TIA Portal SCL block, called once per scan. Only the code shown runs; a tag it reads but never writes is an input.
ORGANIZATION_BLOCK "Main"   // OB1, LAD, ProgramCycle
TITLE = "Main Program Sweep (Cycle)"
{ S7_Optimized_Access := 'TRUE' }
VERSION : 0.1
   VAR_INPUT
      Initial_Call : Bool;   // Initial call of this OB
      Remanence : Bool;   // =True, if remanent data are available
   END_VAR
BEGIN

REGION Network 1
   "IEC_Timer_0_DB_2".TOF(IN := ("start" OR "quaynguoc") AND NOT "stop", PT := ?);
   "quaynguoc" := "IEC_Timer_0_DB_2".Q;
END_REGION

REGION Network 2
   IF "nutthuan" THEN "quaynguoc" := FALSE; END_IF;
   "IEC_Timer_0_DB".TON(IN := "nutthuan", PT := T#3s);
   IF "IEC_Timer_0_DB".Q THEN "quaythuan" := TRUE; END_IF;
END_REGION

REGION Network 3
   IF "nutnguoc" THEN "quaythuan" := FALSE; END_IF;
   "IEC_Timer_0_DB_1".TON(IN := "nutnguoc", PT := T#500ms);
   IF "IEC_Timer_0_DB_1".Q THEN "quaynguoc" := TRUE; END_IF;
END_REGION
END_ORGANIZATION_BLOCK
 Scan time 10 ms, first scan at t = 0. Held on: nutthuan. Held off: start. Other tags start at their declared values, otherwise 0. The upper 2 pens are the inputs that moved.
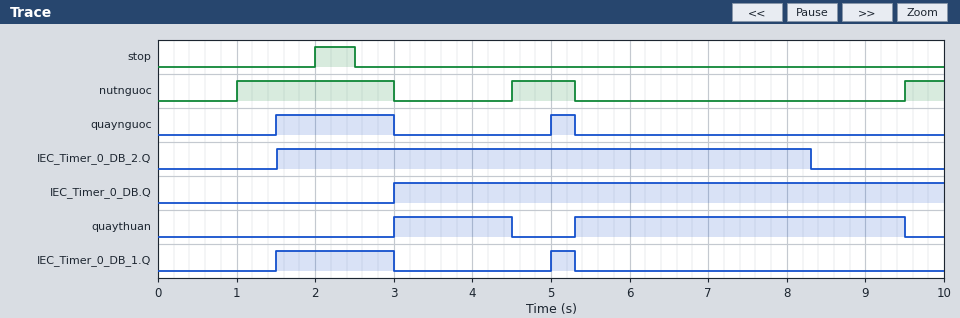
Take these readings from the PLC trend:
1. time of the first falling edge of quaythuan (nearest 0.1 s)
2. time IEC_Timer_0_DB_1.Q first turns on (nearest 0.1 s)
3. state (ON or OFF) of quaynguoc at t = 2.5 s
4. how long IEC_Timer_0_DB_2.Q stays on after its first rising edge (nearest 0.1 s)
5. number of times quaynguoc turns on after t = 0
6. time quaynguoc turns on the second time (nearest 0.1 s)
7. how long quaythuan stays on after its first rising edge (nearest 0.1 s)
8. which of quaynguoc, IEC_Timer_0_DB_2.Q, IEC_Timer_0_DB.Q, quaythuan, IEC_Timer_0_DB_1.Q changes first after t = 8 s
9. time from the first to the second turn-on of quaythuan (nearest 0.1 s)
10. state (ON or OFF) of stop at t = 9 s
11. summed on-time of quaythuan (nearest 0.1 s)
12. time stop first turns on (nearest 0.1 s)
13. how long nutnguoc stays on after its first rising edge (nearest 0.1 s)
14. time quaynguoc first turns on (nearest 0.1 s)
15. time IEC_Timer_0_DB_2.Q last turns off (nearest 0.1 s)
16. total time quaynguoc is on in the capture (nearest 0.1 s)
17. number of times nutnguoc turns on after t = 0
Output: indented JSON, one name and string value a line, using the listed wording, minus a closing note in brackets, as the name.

{
  "time of the first falling edge of quaythuan": "4.5 s",
  "time IEC_Timer_0_DB_1.Q first turns on": "1.5 s",
  "state (ON or OFF) of quaynguoc at t = 2.5 s": "ON",
  "how long IEC_Timer_0_DB_2.Q stays on after its first rising edge": "6.8 s",
  "number of times quaynguoc turns on after t = 0": "2",
  "time quaynguoc turns on the second time": "5.0 s",
  "how long quaythuan stays on after its first rising edge": "1.5 s",
  "which of quaynguoc, IEC_Timer_0_DB_2.Q, IEC_Timer_0_DB.Q, quaythuan, IEC_Timer_0_DB_1.Q changes first after t = 8 s": "IEC_Timer_0_DB_2.Q",
  "time from the first to the second turn-on of quaythuan": "2.3 s",
  "state (ON or OFF) of stop at t = 9 s": "OFF",
  "summed on-time of quaythuan": "5.7 s",
  "time stop first turns on": "2.0 s",
  "how long nutnguoc stays on after its first rising edge": "2.0 s",
  "time quaynguoc first turns on": "1.5 s",
  "time IEC_Timer_0_DB_2.Q last turns off": "8.3 s",
  "total time quaynguoc is on in the capture": "1.8 s",
  "number of times nutnguoc turns on after t = 0": "3"
}
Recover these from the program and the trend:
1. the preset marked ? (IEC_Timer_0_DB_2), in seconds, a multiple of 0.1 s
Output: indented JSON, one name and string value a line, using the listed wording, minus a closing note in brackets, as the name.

{
  "the preset marked ? (IEC_Timer_0_DB_2), in seconds, a multiple of 0.1 s": "3.0 s"
}
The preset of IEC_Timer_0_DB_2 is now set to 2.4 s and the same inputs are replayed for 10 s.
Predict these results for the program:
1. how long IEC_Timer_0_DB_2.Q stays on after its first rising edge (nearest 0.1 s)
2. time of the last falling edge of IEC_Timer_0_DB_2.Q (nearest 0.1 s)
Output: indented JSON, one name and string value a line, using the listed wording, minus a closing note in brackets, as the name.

{
  "how long IEC_Timer_0_DB_2.Q stays on after its first rising edge": "6.2 s",
  "time of the last falling edge of IEC_Timer_0_DB_2.Q": "7.7 s"
}
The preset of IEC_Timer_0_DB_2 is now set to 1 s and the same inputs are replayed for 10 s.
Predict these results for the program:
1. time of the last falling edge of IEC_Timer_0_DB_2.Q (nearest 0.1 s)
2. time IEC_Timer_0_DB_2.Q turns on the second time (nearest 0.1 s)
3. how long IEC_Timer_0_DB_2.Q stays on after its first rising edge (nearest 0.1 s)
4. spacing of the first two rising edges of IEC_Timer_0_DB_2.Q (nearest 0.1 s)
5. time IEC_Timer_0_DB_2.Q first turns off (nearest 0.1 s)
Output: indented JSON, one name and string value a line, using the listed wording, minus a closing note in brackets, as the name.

{
  "time of the last falling edge of IEC_Timer_0_DB_2.Q": "6.3 s",
  "time IEC_Timer_0_DB_2.Q turns on the second time": "5.0 s",
  "how long IEC_Timer_0_DB_2.Q stays on after its first rising edge": "2.5 s",
  "spacing of the first two rising edges of IEC_Timer_0_DB_2.Q": "3.5 s",
  "time IEC_Timer_0_DB_2.Q first turns off": "4.0 s"
}
